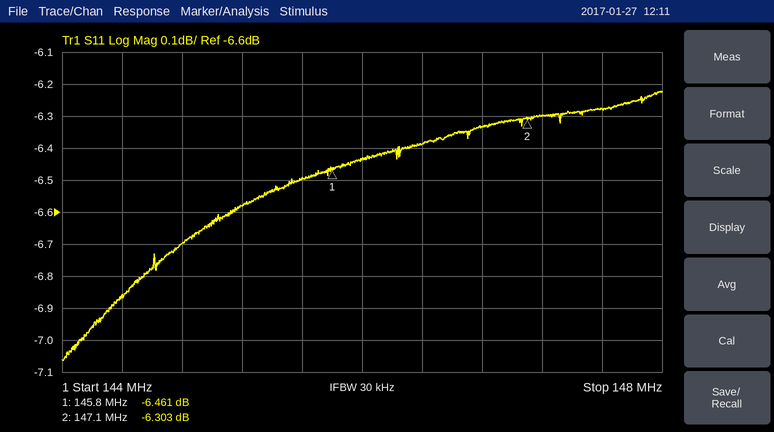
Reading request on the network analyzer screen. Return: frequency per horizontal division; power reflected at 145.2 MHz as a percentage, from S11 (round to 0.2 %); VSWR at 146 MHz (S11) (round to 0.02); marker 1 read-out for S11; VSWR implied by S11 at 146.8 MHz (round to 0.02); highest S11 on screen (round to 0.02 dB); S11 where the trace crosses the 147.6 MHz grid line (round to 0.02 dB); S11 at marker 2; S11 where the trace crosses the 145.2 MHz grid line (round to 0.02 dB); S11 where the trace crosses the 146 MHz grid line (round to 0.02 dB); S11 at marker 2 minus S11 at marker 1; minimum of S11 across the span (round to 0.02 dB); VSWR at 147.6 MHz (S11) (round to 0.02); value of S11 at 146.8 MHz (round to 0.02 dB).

400 kHz
22.0 %
2.82
-6.461 dB
2.86
-6.22 dB
-6.28 dB
-6.303 dB
-6.58 dB
-6.44 dB
0.158 dB
-7.06 dB
2.88
-6.34 dB
